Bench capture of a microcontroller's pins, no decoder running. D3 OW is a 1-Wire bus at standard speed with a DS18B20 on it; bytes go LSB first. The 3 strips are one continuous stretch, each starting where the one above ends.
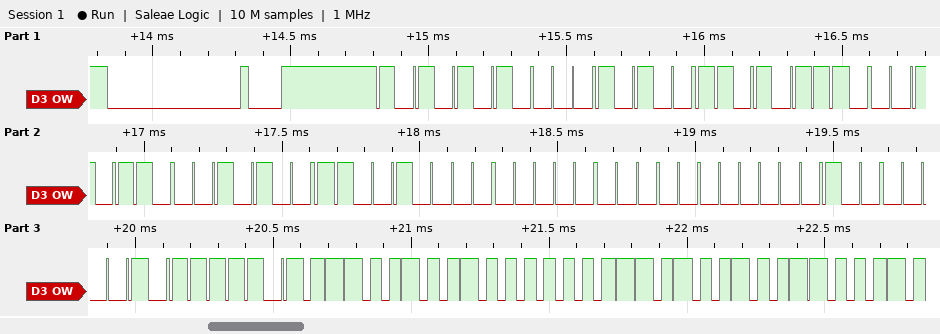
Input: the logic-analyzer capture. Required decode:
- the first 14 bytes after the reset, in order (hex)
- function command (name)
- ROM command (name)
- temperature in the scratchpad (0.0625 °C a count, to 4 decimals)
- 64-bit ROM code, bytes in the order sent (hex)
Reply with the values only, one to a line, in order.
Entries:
55 28 EB 68 94 09 00 00 81 BE 26 01 4B 46
Read Scratchpad
Match ROM
18.3750 °C
28 EB 68 94 09 00 00 81
